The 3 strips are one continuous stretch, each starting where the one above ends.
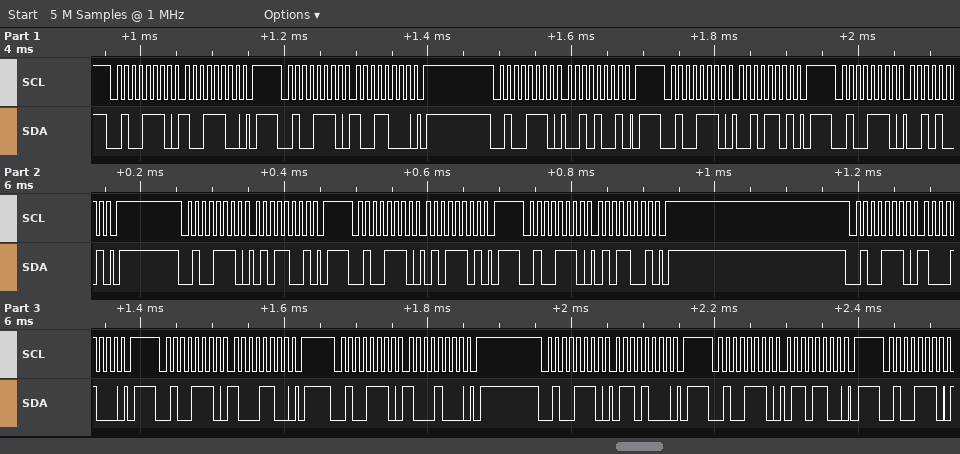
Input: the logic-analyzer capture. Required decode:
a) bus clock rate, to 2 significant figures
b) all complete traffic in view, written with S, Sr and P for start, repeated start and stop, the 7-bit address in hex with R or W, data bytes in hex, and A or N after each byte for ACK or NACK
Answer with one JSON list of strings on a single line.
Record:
["100 kHz", "S 27W A 9C A P S 27W A 98 A P S 27W A 29 A P S 27W A 2D A P S 27W A 29 A P S 27W A 59 A P S 27W A 5D A P S 27W A 59 A P S 27W A 88 A P S 27W A 8C A P S 27W A 88 A P S 27W A 68 A P S 27W A 6C A P S 27W A"]
